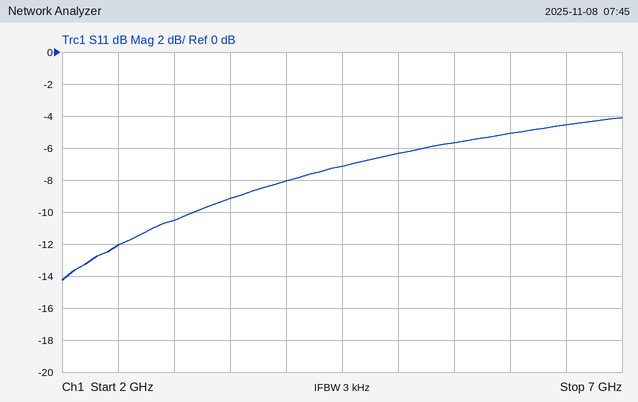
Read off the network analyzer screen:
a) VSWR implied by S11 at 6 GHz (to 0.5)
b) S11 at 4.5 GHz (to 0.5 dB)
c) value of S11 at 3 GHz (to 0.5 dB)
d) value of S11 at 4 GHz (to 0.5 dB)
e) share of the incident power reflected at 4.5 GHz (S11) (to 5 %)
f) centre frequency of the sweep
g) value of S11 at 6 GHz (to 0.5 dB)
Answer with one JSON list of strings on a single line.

["3.5", "-7.0 dB", "-10.5 dB", "-8.0 dB", "20 %", "4.5 GHz", "-5.0 dB"]
